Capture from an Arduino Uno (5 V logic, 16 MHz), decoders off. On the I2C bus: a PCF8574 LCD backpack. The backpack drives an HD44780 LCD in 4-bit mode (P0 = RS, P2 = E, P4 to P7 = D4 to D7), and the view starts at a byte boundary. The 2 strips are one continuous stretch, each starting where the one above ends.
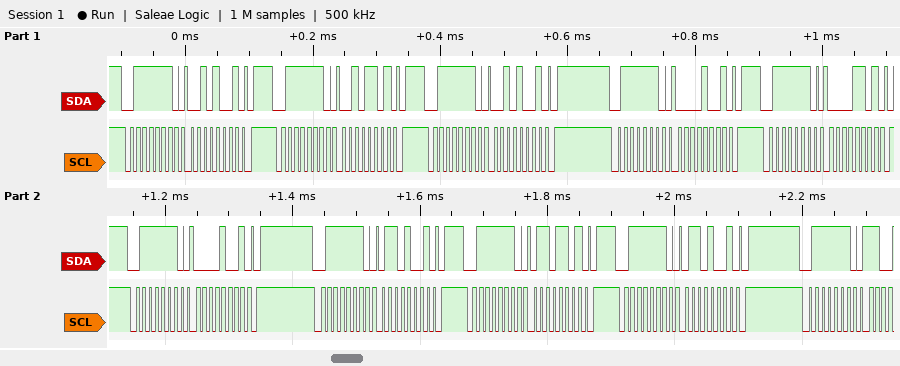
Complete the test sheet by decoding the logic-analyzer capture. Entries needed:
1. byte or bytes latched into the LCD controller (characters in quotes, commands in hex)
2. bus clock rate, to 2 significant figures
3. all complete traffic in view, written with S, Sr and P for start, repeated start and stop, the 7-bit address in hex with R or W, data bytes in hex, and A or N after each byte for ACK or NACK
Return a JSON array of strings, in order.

["' '", "100 kHz", "S 3FW A 29 A P S 3FW A 2D A P S 3FW A 29 A P S 3FW A 09 A P S 3FW A 0D A P S 3FW A 09 A P S 3FW A 69 A P S 3FW A 6D A P S 3FW A 69 A P S 3FW A"]
